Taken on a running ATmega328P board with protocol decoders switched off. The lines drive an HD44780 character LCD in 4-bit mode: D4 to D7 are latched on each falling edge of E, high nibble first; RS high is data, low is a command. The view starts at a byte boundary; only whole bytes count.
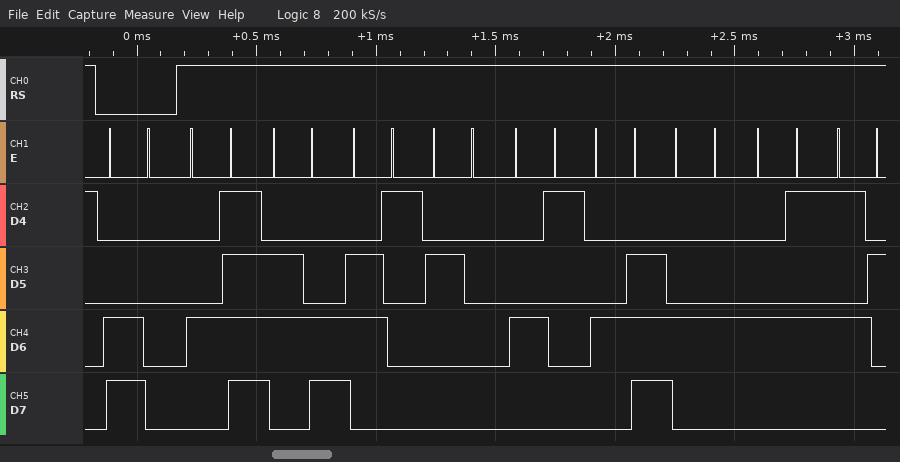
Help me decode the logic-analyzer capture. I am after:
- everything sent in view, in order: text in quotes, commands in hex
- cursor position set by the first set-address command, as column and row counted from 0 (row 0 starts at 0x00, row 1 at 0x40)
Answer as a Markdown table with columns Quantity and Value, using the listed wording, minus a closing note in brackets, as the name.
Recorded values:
| Quantity | Value |
|---|---|
| everything sent in view, in order: text in quotes, commands in hex | 0xC0 "Ola ANDER" |
| cursor position set by the first set-address command, as column and row counted from 0 | column 0, row 1 |
